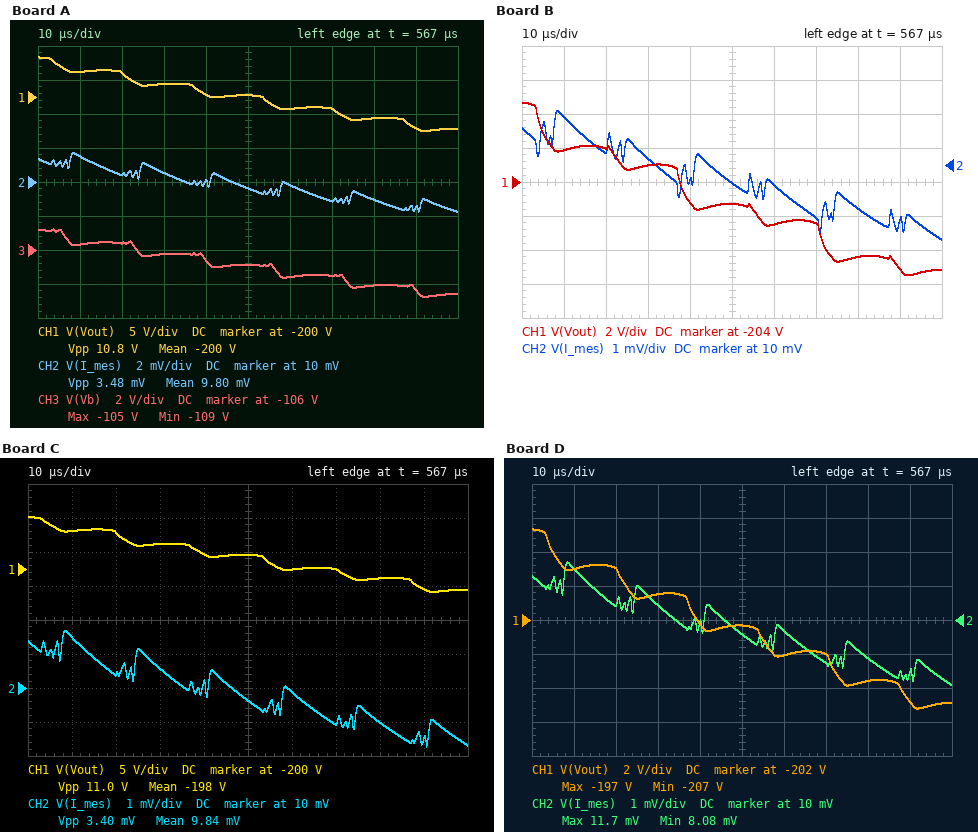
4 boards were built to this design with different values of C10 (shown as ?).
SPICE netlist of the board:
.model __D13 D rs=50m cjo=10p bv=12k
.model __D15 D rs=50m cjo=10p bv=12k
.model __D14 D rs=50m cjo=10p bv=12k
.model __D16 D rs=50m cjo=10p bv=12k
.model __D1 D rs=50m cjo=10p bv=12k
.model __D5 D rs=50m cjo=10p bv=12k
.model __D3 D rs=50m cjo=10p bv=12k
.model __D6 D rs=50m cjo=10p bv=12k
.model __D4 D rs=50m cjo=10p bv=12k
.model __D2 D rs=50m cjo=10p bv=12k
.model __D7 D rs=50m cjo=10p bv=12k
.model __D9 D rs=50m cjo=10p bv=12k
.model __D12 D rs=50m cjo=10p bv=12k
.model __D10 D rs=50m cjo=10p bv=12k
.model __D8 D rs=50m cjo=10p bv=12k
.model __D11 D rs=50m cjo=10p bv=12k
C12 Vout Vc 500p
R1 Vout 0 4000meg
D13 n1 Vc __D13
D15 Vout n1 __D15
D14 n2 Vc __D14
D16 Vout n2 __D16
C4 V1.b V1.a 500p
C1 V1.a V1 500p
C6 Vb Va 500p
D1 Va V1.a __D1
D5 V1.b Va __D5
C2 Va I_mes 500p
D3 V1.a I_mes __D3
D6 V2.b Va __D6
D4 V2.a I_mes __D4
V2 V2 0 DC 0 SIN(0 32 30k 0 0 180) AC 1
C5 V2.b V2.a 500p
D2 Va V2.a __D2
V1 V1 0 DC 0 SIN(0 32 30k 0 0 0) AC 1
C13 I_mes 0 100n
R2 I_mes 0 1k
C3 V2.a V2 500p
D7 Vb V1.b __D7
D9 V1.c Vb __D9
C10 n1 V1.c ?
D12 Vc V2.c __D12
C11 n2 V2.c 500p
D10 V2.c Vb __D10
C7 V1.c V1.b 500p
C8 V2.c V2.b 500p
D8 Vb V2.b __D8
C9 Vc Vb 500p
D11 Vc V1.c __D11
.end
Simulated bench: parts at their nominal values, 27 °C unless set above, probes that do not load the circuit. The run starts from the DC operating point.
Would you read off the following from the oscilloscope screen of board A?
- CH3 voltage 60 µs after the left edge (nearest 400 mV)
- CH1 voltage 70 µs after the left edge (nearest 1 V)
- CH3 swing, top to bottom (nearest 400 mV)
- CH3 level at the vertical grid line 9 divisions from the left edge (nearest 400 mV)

-107.6 V
-202 V
4.0 V
-108.4 V
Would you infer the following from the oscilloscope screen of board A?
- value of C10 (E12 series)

560 pF
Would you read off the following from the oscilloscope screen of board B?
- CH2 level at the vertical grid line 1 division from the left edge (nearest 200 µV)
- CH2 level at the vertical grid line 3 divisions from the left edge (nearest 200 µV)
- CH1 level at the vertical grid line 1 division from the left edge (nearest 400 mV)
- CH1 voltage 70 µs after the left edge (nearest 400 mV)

11.4 mV
10.2 mV
-202.0 V
-206.4 V
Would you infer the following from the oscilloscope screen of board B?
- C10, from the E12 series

180 pF
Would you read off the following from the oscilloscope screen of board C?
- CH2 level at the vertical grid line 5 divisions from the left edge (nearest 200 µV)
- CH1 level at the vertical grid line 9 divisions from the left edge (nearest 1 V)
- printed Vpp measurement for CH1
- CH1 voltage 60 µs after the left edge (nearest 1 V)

9.6 mV
-203 V
11.0 V
-200 V
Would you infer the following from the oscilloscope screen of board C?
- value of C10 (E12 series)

680 pF
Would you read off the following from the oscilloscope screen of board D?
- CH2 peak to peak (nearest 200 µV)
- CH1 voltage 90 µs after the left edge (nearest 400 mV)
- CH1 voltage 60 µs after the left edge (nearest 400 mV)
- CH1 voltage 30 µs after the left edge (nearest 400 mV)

3.6 mV
-206.8 V
-204.0 V
-200.4 V
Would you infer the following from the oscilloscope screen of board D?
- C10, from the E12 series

390 pF
